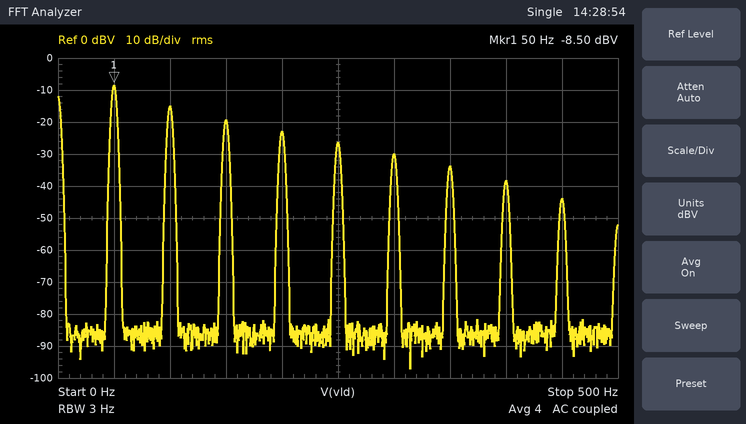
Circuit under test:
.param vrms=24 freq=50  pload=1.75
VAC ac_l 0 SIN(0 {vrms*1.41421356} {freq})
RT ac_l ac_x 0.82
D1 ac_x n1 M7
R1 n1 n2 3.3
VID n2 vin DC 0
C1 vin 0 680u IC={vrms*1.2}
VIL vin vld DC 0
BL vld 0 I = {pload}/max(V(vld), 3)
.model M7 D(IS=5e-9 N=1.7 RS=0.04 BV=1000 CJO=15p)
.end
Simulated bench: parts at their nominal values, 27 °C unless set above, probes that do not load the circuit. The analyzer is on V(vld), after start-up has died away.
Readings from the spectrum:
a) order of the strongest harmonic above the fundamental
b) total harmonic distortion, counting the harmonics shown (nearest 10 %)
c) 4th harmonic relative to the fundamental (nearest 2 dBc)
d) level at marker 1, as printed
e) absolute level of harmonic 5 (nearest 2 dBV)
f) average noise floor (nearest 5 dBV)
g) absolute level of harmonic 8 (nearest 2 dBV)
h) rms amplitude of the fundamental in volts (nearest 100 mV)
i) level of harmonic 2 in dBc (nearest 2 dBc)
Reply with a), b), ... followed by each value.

a) 2
b) 60 %
c) -14 dBc
d) -8.50 dBV
e) -26 dBV
f) -85 dBV
g) -38 dBV
h) 400 mV
i) -6 dBc
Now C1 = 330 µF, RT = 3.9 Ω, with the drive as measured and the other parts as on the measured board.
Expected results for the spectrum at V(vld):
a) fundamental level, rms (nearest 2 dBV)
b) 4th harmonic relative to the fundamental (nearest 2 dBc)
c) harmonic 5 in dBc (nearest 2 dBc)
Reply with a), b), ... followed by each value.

a) -2 dBV
b) -16 dBc
c) -20 dBc
